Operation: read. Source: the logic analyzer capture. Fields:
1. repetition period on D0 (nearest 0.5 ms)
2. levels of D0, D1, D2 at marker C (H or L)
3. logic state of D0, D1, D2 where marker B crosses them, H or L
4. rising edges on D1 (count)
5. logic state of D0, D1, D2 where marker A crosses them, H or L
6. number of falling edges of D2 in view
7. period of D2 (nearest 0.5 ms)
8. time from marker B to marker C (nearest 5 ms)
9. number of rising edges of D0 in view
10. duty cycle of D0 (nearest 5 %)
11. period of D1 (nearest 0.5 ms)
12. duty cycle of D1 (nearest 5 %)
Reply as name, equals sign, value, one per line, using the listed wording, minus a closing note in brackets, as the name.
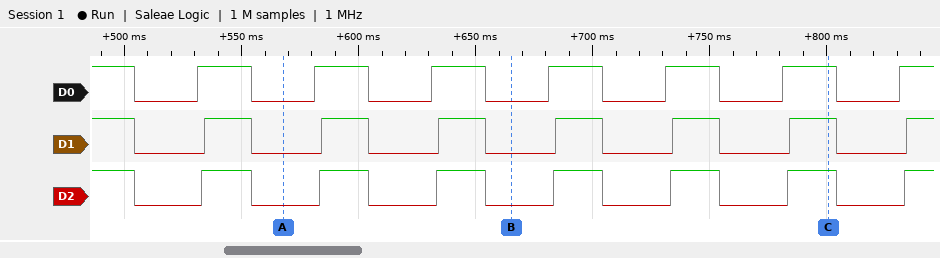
repetition period on D0 = 50 ms
levels of D0, D1, D2 at marker C = D0=H, D1=H, D2=H
logic state of D0, D1, D2 where marker B crosses them, H or L = D0=L, D1=L, D2=L
rising edges on D1 = 7
logic state of D0, D1, D2 where marker A crosses them, H or L = D0=L, D1=L, D2=L
number of falling edges of D2 in view = 7
period of D2 = 50 ms
time from marker B to marker C = 135 ms
number of rising edges of D0 in view = 7
duty cycle of D0 = 45 %
period of D1 = 50 ms
duty cycle of D1 = 40 %
